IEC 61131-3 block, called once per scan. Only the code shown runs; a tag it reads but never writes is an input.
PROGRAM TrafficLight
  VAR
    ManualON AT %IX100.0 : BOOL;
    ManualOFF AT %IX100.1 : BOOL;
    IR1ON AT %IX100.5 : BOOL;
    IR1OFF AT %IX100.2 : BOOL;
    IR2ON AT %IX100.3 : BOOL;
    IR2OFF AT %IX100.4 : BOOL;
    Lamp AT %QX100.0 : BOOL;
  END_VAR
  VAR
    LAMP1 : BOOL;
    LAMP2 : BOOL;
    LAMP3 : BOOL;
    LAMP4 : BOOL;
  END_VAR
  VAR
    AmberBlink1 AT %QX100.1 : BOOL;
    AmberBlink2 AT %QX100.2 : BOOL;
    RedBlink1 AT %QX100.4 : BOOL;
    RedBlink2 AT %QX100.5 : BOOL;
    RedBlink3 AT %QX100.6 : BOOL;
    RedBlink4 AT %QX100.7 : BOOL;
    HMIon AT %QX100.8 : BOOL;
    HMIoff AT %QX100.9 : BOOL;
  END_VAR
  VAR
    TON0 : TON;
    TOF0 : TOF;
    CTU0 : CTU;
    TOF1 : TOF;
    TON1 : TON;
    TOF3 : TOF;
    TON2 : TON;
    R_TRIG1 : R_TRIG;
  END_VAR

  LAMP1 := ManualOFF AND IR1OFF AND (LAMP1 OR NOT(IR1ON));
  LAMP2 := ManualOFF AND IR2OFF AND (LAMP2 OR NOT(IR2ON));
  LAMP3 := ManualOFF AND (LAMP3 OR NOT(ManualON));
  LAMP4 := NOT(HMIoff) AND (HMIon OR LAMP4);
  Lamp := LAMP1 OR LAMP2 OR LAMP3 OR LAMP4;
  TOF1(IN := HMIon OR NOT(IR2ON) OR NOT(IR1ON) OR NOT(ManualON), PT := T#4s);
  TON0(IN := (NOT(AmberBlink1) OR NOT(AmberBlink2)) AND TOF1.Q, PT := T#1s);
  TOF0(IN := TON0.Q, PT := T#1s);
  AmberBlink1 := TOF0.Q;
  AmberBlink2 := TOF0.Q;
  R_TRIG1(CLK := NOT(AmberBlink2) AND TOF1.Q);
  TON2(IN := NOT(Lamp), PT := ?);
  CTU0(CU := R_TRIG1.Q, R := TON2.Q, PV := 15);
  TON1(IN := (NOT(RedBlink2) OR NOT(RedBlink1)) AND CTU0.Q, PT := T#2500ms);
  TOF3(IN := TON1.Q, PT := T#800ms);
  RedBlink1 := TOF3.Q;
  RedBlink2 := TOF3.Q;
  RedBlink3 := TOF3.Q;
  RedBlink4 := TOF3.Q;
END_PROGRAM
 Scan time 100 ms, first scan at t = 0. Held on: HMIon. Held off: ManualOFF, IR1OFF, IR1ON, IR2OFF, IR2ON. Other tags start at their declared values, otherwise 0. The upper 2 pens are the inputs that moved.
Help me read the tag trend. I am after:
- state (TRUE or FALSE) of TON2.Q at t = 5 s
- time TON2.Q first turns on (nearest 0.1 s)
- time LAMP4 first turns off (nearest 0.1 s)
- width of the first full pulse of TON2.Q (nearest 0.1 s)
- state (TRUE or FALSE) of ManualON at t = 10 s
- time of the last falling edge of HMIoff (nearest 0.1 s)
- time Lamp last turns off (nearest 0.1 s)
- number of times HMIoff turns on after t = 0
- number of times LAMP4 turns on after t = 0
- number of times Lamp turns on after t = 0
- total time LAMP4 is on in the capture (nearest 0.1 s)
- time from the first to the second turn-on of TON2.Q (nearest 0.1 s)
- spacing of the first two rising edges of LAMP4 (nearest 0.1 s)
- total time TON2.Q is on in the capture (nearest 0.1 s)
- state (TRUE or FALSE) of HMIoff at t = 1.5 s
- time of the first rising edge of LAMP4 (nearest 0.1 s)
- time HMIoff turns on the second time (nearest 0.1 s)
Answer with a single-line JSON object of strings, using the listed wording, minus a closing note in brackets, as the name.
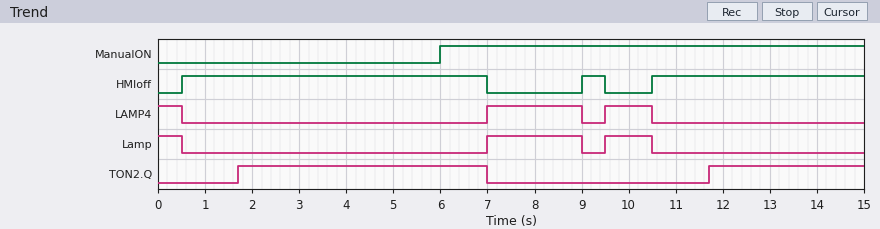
{"state (TRUE or FALSE) of TON2.Q at t = 5 s": "TRUE", "time TON2.Q first turns on": "1.7 s", "time LAMP4 first turns off": "0.5 s", "width of the first full pulse of TON2.Q": "5.3 s", "state (TRUE or FALSE) of ManualON at t = 10 s": "TRUE", "time of the last falling edge of HMIoff": "9.5 s", "time Lamp last turns off": "10.5 s", "number of times HMIoff turns on after t = 0": "3", "number of times LAMP4 turns on after t = 0": "2", "number of times Lamp turns on after t = 0": "2", "total time LAMP4 is on in the capture": "3.5 s", "time from the first to the second turn-on of TON2.Q": "10.0 s", "spacing of the first two rising edges of LAMP4": "2.5 s", "total time TON2.Q is on in the capture": "8.6 s", "state (TRUE or FALSE) of HMIoff at t = 1.5 s": "TRUE", "time of the first rising edge of LAMP4": "7.0 s", "time HMIoff turns on the second time": "9.0 s"}
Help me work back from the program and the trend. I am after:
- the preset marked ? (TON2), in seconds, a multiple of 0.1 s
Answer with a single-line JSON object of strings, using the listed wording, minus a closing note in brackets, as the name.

{"the preset marked ? (TON2), in seconds, a multiple of 0.1 s": "1.2 s"}
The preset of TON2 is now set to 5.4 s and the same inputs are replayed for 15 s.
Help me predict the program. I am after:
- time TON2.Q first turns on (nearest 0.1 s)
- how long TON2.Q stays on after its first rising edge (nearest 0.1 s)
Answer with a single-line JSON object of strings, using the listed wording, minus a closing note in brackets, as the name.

{"time TON2.Q first turns on": "5.9 s", "how long TON2.Q stays on after its first rising edge": "1.1 s"}
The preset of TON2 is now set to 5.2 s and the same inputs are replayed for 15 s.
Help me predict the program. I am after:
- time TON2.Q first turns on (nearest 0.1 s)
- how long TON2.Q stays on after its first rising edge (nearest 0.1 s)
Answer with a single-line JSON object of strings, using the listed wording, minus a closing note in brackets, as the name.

{"time TON2.Q first turns on": "5.7 s", "how long TON2.Q stays on after its first rising edge": "1.3 s"}
